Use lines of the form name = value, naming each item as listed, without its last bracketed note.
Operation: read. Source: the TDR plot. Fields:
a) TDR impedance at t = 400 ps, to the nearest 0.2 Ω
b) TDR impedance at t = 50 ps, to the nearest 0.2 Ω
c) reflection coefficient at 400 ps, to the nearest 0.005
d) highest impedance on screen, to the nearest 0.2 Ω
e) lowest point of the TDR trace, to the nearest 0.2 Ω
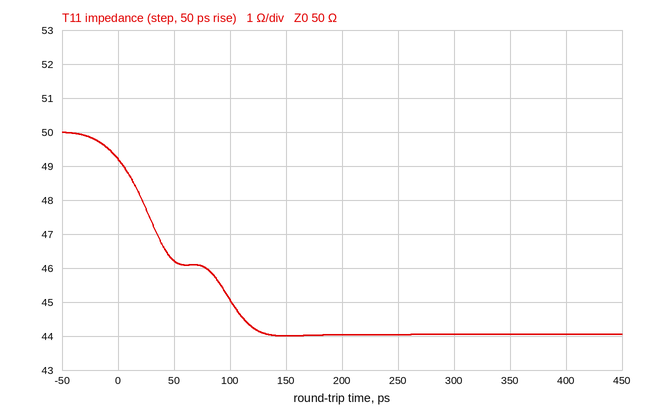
TDR impedance at t = 400 ps, to the nearest 0.2 Ω = 44.0 Ω
TDR impedance at t = 50 ps, to the nearest 0.2 Ω = 46.2 Ω
reflection coefficient at 400 ps, to the nearest 0.005 = -0.065
highest impedance on screen, to the nearest 0.2 Ω = 50.0 Ω
lowest point of the TDR trace, to the nearest 0.2 Ω = 44.0 Ω
